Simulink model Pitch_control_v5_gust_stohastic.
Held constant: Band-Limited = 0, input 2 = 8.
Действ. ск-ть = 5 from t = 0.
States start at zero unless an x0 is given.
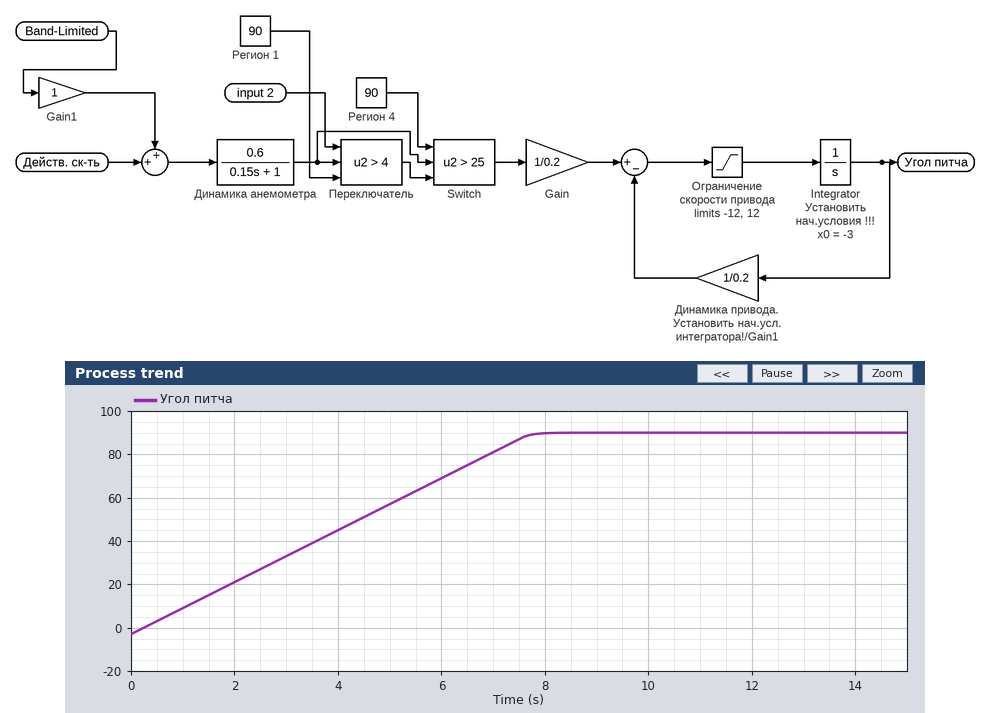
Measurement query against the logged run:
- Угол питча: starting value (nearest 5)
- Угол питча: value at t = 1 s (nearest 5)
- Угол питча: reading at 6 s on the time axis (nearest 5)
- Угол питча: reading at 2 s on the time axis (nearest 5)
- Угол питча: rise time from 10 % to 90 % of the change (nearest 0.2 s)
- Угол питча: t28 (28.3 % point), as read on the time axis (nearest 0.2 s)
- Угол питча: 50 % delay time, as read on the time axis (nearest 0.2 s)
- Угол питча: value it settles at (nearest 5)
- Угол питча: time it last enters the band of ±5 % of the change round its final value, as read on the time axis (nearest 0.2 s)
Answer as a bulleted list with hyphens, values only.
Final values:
- -5
- 10
- 70
- 20
- 6.2 s
- 2.2 s
- 3.8 s
- 90
- 7.4 s
